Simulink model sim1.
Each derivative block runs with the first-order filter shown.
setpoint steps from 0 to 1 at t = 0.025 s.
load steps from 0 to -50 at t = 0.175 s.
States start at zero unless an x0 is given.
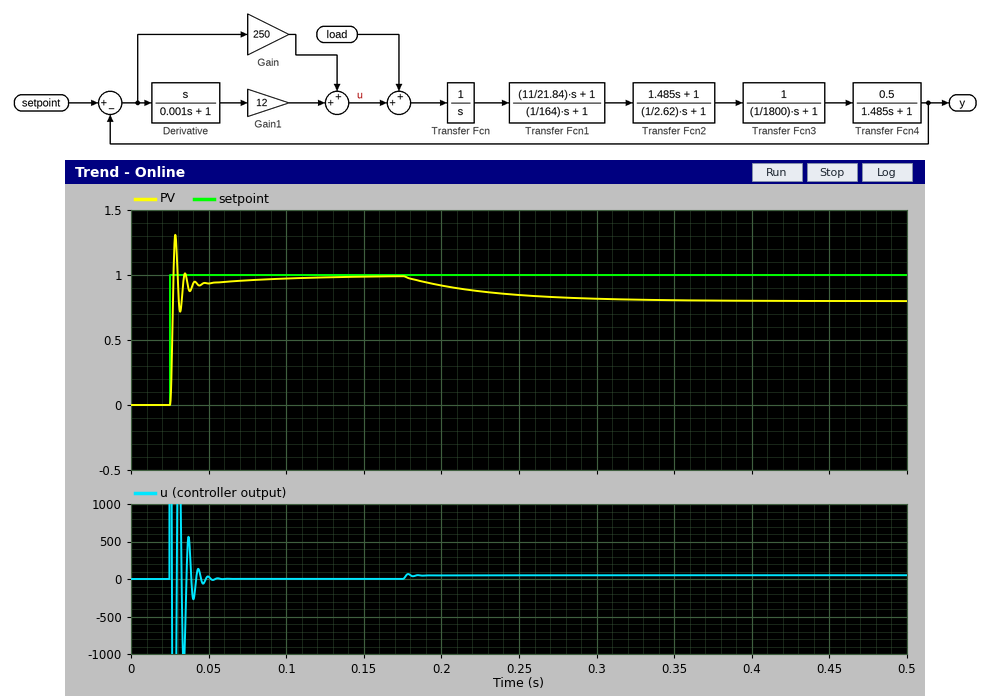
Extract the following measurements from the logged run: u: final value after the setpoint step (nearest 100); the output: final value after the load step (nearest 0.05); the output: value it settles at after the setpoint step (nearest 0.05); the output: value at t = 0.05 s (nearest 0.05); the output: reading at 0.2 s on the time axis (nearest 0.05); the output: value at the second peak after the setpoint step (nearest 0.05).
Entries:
0
0.80
1.00
0.95
0.90
1.00
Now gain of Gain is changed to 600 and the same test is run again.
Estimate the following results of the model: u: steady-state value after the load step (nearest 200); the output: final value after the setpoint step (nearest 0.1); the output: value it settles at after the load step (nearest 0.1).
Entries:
0
1.0
0.9
